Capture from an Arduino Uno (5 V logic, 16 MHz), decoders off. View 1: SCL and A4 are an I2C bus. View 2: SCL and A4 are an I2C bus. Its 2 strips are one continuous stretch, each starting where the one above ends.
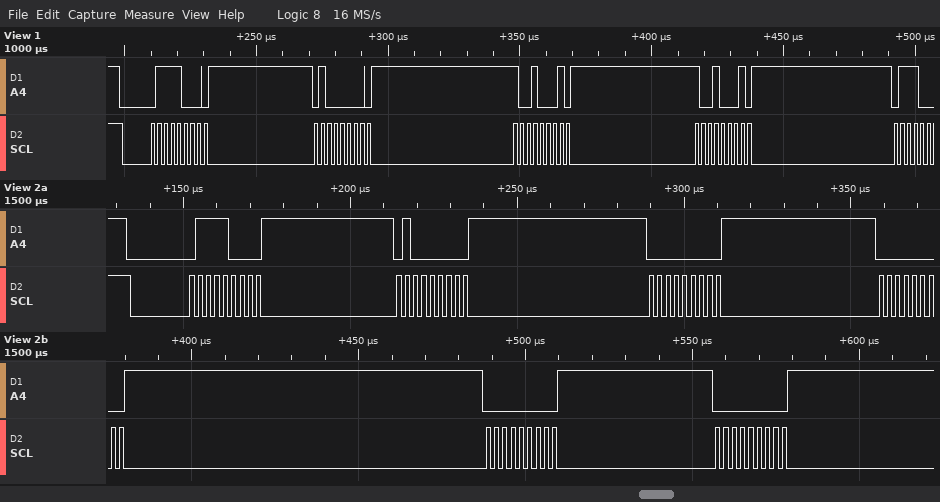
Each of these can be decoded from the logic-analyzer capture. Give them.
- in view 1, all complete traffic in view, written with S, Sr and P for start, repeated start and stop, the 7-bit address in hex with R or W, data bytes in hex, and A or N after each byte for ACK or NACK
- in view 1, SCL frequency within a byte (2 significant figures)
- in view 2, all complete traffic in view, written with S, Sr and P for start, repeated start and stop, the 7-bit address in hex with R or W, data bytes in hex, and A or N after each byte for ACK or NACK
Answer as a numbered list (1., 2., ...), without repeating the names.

1. S 3CW A 40 A 91 A 91 A
2. 400 kHz
3. S 3CW A 40 A 00 A 00 A 00 A 00 A
